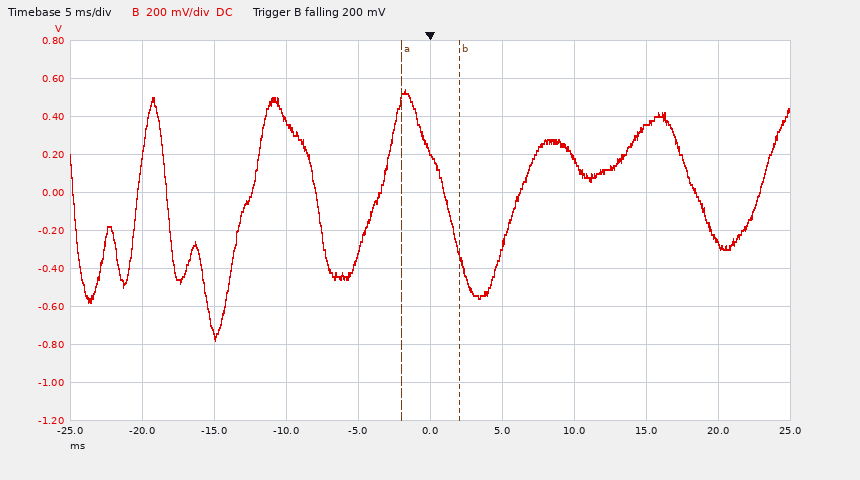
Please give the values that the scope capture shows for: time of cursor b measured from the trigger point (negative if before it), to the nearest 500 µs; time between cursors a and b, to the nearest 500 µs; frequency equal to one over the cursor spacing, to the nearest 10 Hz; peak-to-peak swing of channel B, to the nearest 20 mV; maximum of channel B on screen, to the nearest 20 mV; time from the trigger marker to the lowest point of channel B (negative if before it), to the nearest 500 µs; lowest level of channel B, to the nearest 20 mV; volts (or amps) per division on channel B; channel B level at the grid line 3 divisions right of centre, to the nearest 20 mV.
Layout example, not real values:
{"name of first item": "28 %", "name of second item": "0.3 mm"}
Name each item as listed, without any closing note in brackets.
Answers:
{"time of cursor b measured from the trigger point (negative if before it), to the nearest 500 µs": "+2.0 ms", "time between cursors a and b, to the nearest 500 µs": "4.0 ms", "frequency equal to one over the cursor spacing, to the nearest 10 Hz": "250 Hz", "peak-to-peak swing of channel B, to the nearest 20 mV": "1.32 V", "maximum of channel B on screen, to the nearest 20 mV": "540 mV", "time from the trigger marker to the lowest point of channel B (negative if before it), to the nearest 500 µs": "-15.0 ms", "lowest level of channel B, to the nearest 20 mV": "-780 mV", "volts (or amps) per division on channel B": "200 mV", "channel B level at the grid line 3 divisions right of centre, to the nearest 20 mV": "340 mV"}
